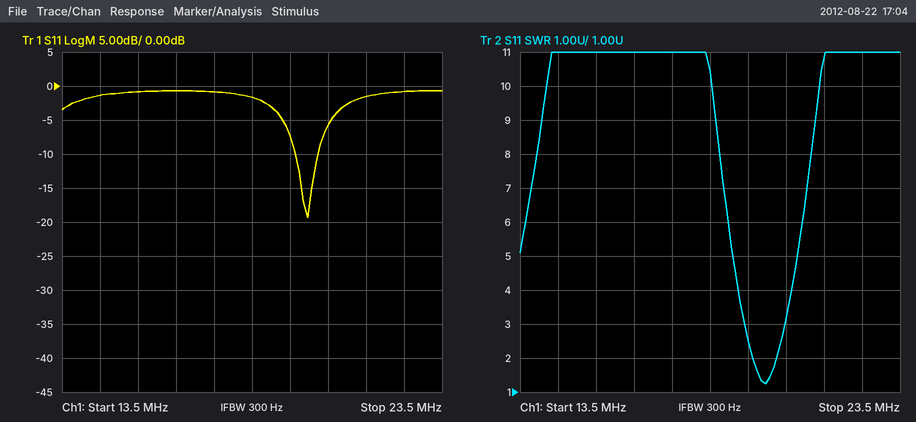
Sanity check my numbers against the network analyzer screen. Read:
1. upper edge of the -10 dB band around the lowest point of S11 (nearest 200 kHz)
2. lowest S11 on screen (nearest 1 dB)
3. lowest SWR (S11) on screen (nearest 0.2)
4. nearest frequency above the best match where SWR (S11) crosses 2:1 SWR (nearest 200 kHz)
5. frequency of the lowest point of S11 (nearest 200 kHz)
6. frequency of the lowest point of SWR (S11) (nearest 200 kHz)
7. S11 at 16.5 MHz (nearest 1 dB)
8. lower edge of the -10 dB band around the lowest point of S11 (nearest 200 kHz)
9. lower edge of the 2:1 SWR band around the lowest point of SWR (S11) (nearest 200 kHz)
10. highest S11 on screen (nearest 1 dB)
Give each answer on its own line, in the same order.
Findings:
20.2 MHz
-19 dB
1.2
20.2 MHz
20.0 MHz
20.0 MHz
-1 dB
19.6 MHz
19.6 MHz
-1 dB
